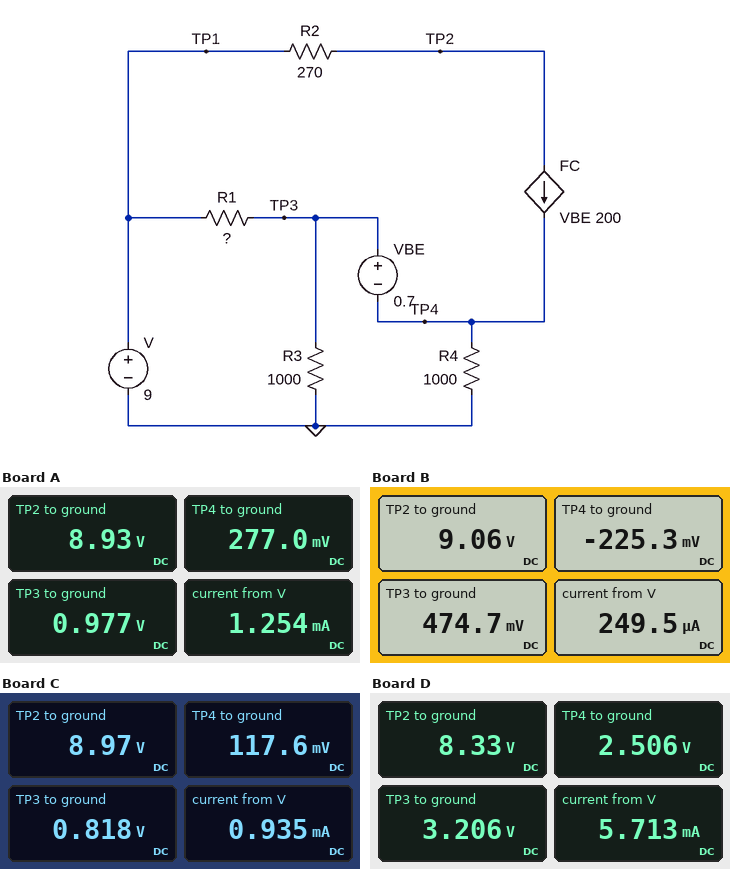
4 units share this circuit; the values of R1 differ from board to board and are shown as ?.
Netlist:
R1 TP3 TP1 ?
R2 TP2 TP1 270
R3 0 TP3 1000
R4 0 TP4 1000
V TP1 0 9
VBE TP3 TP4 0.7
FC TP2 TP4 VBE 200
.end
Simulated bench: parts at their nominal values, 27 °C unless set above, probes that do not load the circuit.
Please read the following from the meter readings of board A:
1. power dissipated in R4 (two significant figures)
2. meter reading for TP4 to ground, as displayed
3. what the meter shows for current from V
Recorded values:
77 µW
277.0 mV
1.254 mA
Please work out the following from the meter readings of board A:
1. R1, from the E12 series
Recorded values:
8.2 kΩ
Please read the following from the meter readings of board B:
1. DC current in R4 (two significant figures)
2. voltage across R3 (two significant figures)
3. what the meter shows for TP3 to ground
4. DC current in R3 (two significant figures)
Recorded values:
230 µA
470 mV
474.7 mV
470 µA
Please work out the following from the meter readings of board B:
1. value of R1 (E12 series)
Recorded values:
18 kΩ
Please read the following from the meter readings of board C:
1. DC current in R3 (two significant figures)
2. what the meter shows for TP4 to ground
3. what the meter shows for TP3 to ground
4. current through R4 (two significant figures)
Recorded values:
820 µA
117.6 mV
0.818 V
120 µA
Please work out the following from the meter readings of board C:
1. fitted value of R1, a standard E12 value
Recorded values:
10 kΩ
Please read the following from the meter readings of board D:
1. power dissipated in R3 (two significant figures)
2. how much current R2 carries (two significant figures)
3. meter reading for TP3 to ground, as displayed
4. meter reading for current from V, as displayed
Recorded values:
10 mW
2.5 mA
3.206 V
5.713 mA
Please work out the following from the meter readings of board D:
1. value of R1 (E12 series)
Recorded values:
1.8 kΩ
